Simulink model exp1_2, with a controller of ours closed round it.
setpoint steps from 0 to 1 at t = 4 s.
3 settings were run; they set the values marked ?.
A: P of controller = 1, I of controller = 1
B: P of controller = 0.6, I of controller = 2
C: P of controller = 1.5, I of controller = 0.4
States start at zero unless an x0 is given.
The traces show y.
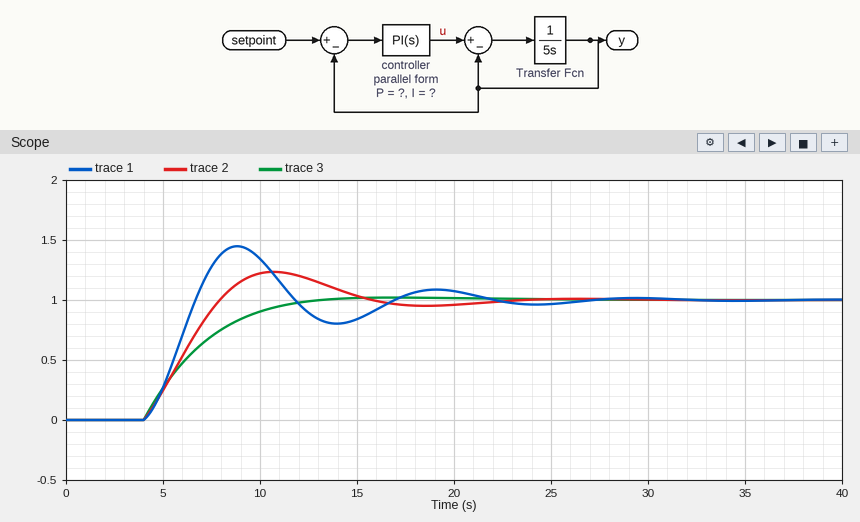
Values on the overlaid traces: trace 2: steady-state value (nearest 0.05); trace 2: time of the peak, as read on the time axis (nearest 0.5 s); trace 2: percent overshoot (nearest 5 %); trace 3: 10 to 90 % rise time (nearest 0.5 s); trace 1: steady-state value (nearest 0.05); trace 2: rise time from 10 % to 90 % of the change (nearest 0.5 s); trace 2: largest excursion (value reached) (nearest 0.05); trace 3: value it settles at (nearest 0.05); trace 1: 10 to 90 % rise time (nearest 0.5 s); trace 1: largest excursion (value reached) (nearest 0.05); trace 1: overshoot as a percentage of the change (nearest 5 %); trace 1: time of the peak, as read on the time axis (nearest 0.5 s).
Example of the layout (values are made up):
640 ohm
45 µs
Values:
1.00
10.5 s
25 %
5.5 s
1.00
3.0 s
1.25
1.00
2.0 s
1.45
45 %
9.0 s
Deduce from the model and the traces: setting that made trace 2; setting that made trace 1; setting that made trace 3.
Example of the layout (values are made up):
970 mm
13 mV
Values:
A
B
C
